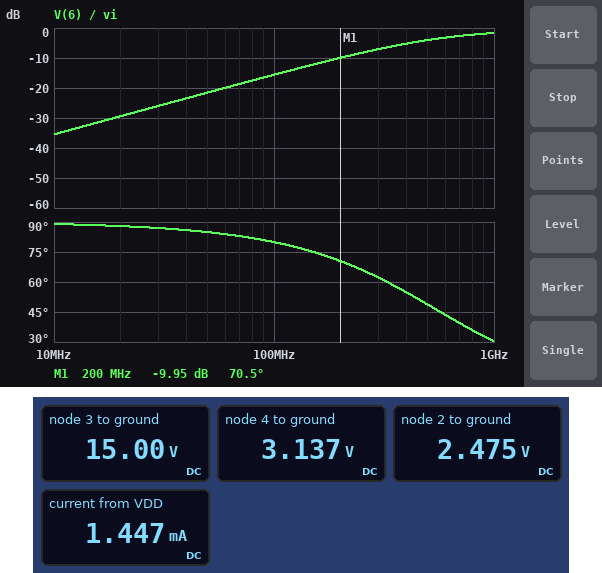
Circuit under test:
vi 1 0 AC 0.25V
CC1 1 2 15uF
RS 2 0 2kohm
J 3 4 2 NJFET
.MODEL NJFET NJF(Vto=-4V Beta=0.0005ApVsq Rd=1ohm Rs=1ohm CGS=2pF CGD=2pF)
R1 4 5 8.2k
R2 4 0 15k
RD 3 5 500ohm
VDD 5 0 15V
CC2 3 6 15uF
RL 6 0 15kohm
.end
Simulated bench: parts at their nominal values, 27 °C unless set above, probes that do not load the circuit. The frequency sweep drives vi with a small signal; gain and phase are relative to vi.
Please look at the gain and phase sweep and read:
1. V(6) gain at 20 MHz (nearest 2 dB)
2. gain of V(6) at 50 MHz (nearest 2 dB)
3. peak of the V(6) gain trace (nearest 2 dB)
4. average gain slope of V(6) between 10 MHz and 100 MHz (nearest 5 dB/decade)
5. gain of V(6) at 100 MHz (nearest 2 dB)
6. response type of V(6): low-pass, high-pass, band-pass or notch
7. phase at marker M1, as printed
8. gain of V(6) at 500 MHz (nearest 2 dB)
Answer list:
-30 dB
-22 dB
-2 dB
20 dB/decade
-16 dB
high-pass
70.5 deg
-4 dB
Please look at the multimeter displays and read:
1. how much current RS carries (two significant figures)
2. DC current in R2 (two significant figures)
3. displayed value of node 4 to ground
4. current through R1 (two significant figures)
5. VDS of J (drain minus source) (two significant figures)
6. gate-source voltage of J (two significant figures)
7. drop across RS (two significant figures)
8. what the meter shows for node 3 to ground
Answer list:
1.2 mA
210 µA
3.137 V
1.4 mA
13 V
660 mV
2.5 V
15.00 V
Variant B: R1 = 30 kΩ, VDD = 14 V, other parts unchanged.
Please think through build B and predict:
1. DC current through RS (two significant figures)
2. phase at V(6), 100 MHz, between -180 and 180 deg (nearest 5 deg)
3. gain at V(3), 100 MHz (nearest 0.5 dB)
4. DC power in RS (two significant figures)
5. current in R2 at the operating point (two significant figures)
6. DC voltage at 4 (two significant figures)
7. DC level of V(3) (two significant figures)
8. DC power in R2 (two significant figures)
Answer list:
340 µA
80 deg
-16.0 dB
230 µW
87 µA
1.3 V
14 V
110 µW
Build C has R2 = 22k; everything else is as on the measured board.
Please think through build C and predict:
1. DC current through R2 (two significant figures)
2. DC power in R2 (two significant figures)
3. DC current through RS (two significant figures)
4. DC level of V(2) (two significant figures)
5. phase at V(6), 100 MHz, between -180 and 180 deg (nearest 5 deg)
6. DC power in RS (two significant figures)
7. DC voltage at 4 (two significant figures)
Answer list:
150 µA
480 µW
1.3 mA
2.6 V
80 deg
3.3 mW
3.2 V
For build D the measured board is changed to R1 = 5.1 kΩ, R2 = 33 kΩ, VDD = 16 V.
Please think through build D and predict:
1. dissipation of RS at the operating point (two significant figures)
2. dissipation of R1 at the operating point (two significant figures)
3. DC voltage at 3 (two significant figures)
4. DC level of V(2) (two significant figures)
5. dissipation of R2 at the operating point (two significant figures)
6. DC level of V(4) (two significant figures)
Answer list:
8.4 mW
25 mW
16 V
4.1 V
690 µW
4.8 V
